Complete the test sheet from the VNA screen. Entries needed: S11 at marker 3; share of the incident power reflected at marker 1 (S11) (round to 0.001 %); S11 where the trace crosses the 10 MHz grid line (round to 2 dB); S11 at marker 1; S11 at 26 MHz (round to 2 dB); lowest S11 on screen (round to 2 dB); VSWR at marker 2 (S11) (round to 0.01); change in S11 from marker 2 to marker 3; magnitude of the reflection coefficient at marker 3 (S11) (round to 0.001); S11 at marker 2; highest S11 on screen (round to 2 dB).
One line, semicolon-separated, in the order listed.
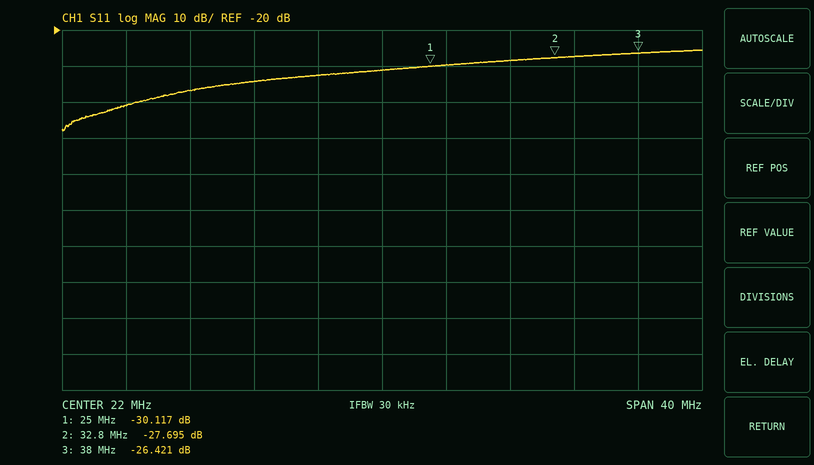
-26.421 dB; 0.097 %; -36 dB; -30.117 dB; -30 dB; -48 dB; 1.09; 1.274 dB; 0.048; -27.695 dB; -26 dB
